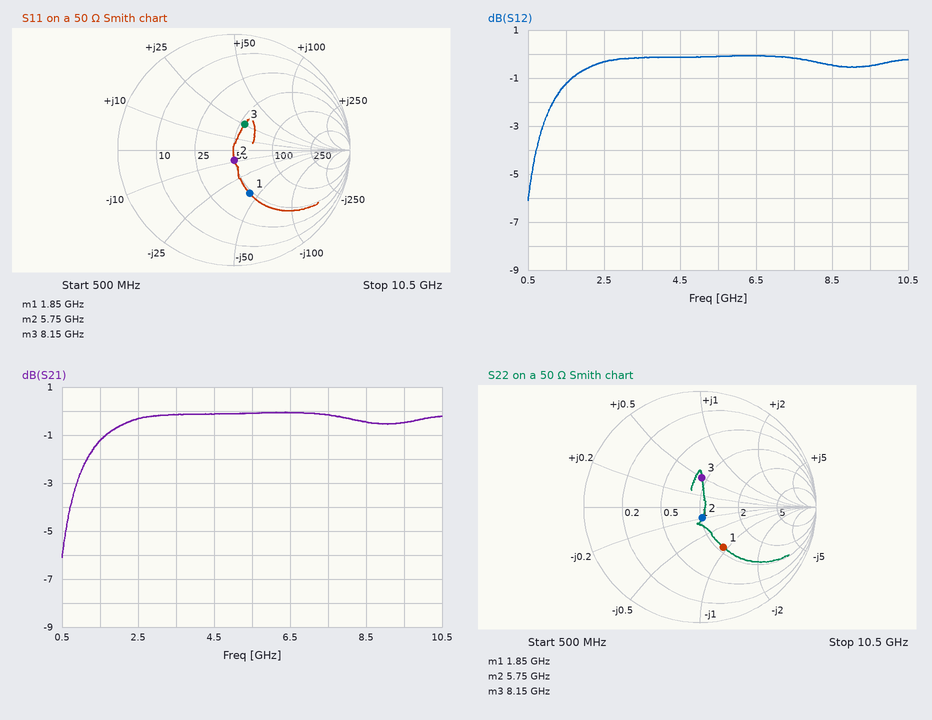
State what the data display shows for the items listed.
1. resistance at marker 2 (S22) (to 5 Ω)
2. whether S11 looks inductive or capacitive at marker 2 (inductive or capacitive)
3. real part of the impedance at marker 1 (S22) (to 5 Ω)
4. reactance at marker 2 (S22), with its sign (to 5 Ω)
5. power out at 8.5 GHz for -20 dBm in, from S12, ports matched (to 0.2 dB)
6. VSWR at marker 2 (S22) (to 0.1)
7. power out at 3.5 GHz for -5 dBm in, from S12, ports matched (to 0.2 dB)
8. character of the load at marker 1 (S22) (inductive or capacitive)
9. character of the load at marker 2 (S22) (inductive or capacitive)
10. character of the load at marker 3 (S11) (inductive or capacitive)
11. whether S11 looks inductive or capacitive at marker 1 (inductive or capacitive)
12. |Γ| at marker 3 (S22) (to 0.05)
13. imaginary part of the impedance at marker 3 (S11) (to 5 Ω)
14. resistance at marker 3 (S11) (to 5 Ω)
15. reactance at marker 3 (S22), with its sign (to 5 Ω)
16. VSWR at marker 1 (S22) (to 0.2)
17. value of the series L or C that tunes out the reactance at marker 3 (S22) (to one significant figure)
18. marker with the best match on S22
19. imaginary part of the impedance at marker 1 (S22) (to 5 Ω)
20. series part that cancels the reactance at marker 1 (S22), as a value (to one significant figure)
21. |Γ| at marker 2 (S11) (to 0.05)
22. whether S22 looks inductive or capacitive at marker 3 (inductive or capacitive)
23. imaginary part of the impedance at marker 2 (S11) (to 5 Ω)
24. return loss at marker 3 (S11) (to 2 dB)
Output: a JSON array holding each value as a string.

["50 Ω", "capacitive", "55 Ω", "-10 Ω", "-20.4 dBm", "1.2", "-5.2 dBm", "capacitive", "capacitive", "inductive", "capacitive", "0.25", "+25 Ω", "55 Ω", "+25 Ω", "2.4", "800 fF", "marker 2", "-45 Ω", "4 nH", "0.10", "inductive", "-10 Ω", "12 dB"]
